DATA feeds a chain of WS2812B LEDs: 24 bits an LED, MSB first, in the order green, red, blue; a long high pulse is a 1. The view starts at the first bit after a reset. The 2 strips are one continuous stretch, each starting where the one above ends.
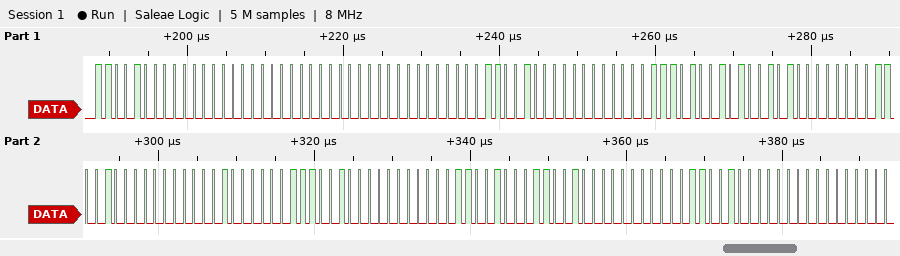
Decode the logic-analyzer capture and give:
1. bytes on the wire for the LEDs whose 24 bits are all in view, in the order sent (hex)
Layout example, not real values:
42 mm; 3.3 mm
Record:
C8 00 00 00 00 C8 00 74 A5 00 C8 00 81 C8 00 C8 C8 00
